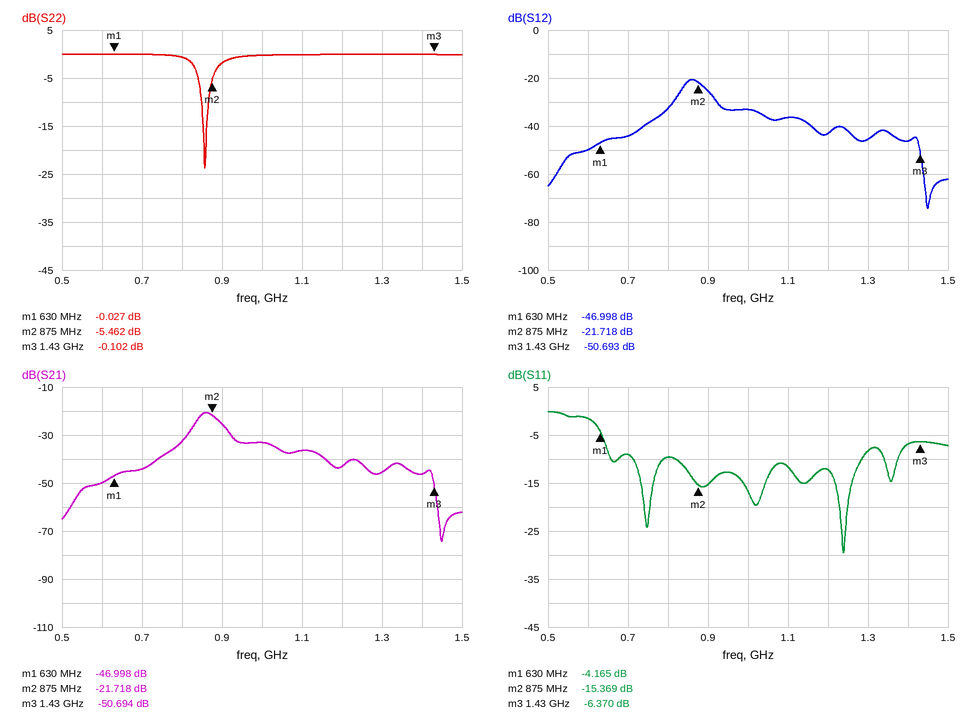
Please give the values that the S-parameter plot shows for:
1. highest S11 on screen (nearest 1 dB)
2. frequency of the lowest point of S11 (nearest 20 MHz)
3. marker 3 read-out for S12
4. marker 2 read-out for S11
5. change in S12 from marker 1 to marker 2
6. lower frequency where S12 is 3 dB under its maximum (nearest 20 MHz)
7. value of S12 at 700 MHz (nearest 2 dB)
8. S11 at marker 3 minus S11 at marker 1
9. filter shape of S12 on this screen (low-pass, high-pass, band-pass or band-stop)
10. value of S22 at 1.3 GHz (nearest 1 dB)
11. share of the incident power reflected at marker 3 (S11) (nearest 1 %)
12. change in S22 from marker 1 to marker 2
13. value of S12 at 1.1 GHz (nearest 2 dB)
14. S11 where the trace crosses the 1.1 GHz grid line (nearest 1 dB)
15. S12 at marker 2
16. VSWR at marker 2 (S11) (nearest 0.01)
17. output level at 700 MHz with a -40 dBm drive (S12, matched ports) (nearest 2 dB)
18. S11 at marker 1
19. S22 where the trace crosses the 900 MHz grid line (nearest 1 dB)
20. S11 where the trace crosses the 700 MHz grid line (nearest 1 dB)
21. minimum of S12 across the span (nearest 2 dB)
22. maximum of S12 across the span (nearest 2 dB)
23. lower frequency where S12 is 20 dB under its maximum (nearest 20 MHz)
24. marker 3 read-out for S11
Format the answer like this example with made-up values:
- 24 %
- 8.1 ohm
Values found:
- 0 dB
- 1.24 GHz
- -50.693 dB
- -15.369 dB
- 25.280 dB
- 840 MHz
- -44 dB
- -2.205 dB
- band-pass
- 0 dB
- 23 %
- -5.435 dB
- -36 dB
- -12 dB
- -21.718 dB
- 1.41
- -84 dBm
- -4.165 dB
- -2 dB
- -9 dB
- -74 dB
- -20 dB
- 740 MHz
- -6.370 dB
